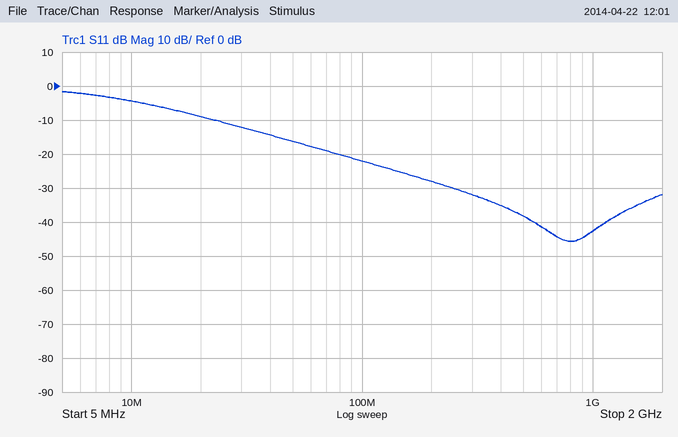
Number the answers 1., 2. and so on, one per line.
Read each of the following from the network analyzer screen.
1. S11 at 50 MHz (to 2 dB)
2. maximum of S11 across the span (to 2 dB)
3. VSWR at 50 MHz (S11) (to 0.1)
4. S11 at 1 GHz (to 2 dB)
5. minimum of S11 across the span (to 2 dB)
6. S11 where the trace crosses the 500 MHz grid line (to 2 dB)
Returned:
1. -16 dB
2. -2 dB
3. 1.4
4. -42 dB
5. -46 dB
6. -38 dB
